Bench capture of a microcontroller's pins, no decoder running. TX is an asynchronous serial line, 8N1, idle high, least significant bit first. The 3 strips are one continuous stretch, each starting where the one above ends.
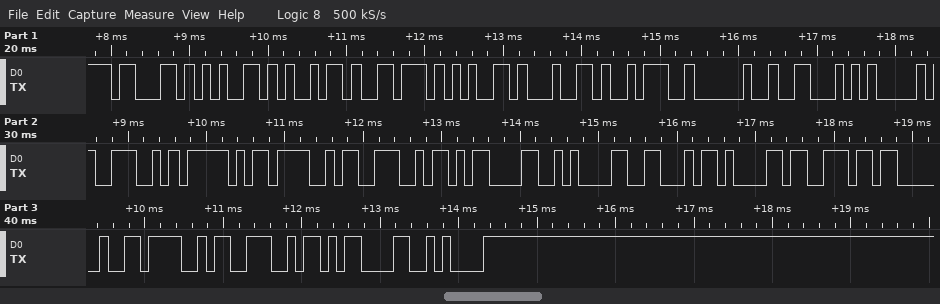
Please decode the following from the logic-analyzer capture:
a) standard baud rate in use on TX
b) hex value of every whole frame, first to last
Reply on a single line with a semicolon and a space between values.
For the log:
9600 baud; 63 65 69 76 65 64 3A 20 46 41 4E 5F 4F 4E 0D 0A 46 61 6E 20 4F 4E 0D 0A
